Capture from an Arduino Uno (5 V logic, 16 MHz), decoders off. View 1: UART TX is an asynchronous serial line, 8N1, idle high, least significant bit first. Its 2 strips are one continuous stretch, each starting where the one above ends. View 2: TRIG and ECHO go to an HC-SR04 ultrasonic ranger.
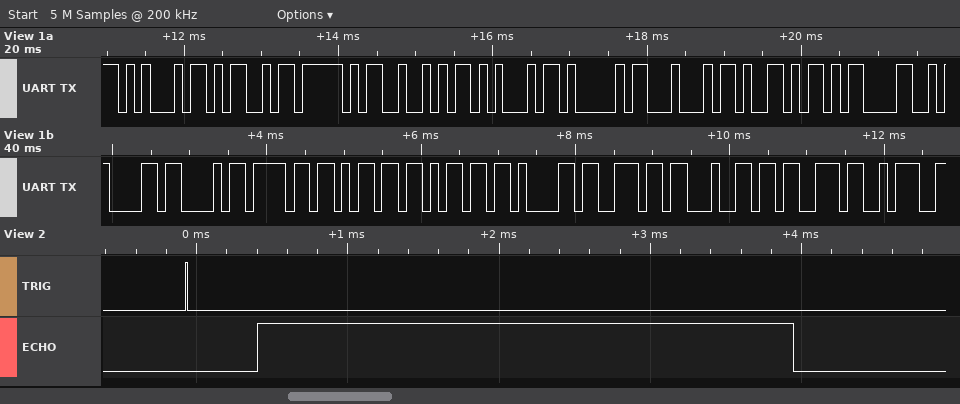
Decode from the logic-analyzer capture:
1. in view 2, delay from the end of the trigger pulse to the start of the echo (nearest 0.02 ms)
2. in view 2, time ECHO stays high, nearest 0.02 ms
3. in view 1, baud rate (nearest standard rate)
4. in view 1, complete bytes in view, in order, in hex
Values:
0.46 ms
3.54 ms
9600 baud
0x45 0x4D 0x5F 0x52 0x45 0x41 0x44 0x59 0x0D 0x0A 0x43 0x6F 0x6D 0x6D 0x61 0x6E 0x64 0x73 0x3A
